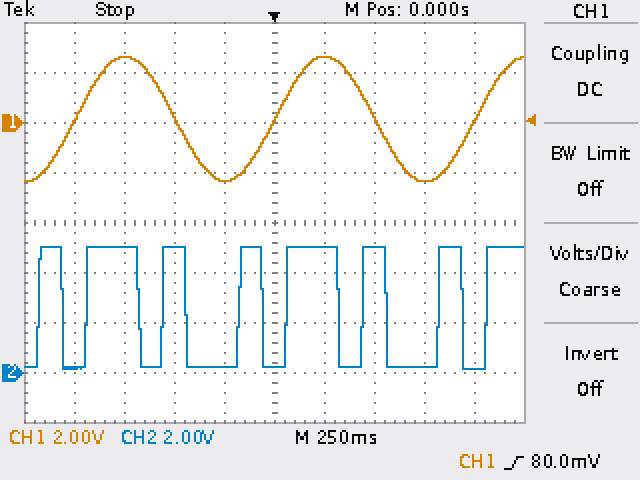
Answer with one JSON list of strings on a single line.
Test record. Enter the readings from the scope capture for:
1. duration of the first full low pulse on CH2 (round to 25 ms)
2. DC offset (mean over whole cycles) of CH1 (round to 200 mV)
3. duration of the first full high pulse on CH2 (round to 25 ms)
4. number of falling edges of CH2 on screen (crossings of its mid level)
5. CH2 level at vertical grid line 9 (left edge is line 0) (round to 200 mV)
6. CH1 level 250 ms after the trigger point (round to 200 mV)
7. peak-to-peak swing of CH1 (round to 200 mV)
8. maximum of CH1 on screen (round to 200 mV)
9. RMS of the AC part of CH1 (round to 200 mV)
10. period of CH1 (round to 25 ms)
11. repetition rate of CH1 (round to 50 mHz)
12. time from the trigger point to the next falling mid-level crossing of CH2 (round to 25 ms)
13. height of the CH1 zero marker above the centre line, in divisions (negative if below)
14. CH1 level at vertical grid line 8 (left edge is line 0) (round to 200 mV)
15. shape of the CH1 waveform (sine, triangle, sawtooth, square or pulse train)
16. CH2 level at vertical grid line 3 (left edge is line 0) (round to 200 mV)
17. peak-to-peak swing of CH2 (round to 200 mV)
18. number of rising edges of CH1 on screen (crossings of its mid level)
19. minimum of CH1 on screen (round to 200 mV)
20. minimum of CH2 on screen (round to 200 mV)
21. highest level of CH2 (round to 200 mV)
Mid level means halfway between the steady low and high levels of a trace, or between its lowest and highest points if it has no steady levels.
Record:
["125 ms", "200 mV", "125 ms", "7", "200 mV", "2.6 V", "5.0 V", "2.6 V", "1.8 V", "1.000 s", "1.00 Hz", "325 ms", "+2.0 div", "-2.4 V", "sine", "5.0 V", "4.8 V", "3", "-2.4 V", "200 mV", "5.0 V"]
